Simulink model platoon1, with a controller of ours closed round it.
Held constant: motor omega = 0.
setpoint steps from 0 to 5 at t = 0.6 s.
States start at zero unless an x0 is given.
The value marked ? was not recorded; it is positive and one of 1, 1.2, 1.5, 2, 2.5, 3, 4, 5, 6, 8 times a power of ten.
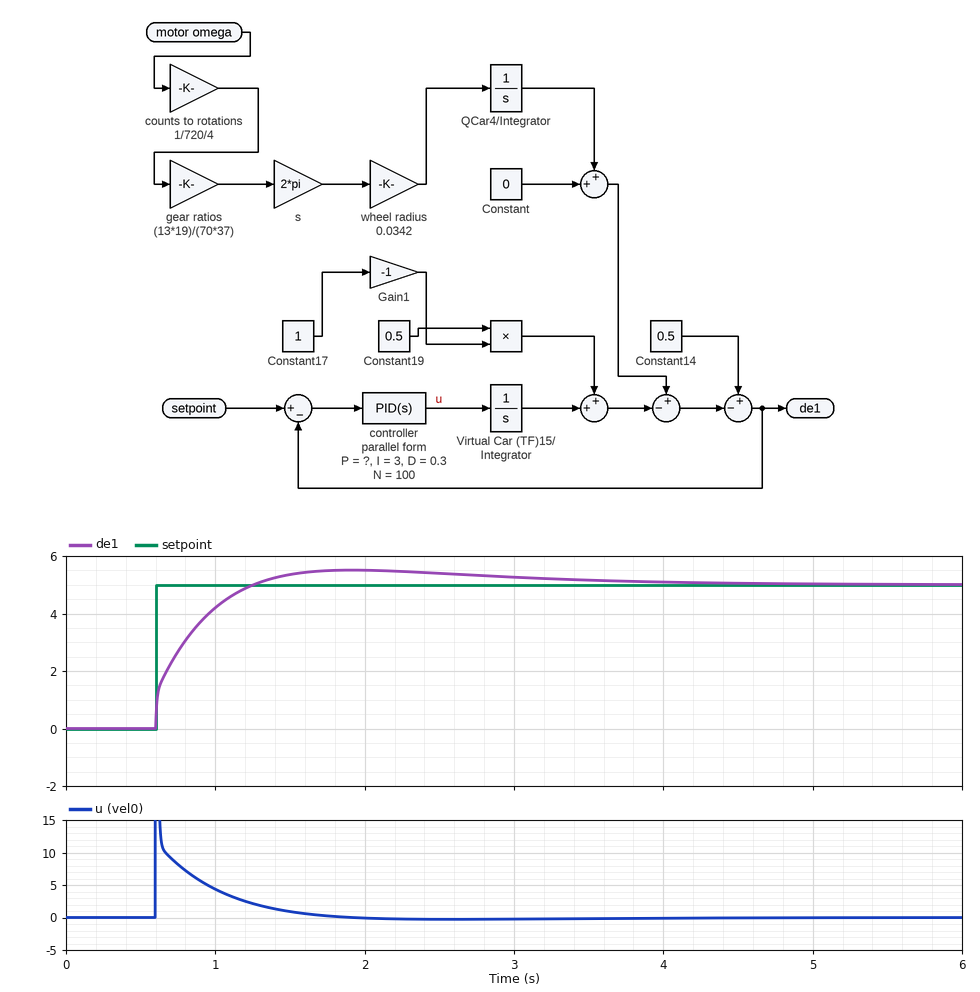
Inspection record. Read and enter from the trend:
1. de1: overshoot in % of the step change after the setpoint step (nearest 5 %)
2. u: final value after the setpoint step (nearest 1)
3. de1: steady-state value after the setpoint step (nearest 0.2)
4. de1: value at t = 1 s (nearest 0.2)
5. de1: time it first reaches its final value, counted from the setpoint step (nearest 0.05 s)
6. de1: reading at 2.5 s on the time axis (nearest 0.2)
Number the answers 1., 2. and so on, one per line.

1. 10 %
2. 0
3. 5.0
4. 4.2
5. 0.65 s
6. 5.4
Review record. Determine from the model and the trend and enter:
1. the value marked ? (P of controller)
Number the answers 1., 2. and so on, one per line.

1. 4
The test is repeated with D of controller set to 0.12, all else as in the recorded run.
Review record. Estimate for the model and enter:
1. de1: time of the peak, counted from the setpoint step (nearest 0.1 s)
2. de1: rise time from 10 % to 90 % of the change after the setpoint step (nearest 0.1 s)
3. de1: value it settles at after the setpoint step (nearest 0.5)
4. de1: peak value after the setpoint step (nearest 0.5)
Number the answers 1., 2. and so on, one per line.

1. 1.2 s
2. 0.4 s
3. 5.0
4. 5.5
